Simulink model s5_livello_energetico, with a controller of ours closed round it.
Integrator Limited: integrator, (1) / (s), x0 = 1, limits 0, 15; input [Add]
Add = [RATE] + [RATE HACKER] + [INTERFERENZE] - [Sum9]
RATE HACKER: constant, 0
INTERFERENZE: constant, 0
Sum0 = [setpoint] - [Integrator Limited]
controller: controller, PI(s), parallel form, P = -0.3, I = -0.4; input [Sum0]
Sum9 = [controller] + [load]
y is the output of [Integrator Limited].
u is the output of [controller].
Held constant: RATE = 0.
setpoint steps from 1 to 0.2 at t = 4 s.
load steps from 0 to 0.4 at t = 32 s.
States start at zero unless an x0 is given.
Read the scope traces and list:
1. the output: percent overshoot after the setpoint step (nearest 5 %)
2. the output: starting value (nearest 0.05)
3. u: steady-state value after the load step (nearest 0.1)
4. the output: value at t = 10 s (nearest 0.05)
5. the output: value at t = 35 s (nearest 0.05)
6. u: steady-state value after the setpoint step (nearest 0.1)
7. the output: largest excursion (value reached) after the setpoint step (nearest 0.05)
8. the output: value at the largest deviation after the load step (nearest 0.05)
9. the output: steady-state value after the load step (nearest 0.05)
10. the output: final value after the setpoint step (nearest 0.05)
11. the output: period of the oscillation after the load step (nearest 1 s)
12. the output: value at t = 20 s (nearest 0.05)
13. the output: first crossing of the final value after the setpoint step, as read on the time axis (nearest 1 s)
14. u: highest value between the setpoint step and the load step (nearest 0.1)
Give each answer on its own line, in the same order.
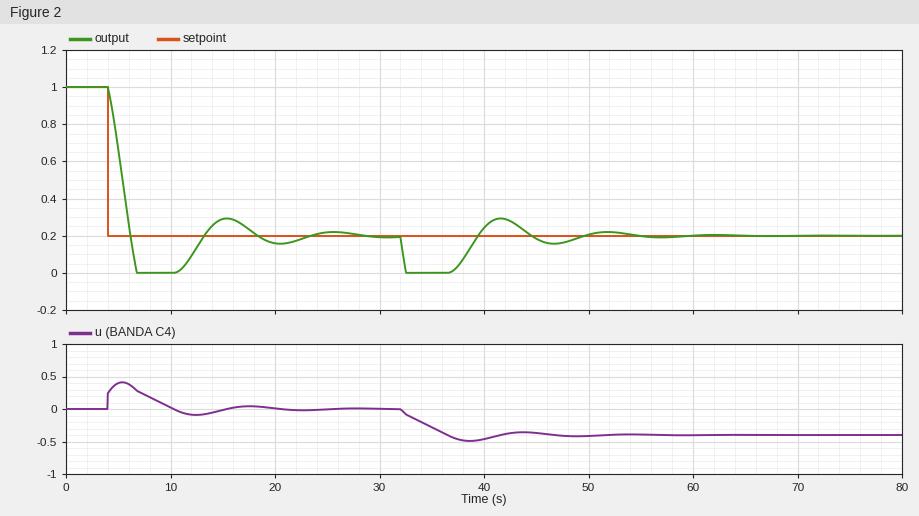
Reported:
25 %
1.00
-0.4
0.00
0.00
0.0
0.00
0.00
0.20
0.20
12 s
0.15
6 s
0.4
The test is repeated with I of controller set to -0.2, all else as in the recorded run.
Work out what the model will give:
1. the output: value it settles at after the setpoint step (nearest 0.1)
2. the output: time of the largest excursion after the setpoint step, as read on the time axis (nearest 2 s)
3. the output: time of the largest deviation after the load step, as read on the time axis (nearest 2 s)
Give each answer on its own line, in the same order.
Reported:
0.2
8 s
32 s
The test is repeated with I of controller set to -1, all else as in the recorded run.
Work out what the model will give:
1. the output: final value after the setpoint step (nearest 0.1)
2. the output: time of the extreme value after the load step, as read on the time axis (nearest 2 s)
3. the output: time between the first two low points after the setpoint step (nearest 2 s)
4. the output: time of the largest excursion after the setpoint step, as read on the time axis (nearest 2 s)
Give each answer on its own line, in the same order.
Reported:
0.2
32 s
8 s
6 s
